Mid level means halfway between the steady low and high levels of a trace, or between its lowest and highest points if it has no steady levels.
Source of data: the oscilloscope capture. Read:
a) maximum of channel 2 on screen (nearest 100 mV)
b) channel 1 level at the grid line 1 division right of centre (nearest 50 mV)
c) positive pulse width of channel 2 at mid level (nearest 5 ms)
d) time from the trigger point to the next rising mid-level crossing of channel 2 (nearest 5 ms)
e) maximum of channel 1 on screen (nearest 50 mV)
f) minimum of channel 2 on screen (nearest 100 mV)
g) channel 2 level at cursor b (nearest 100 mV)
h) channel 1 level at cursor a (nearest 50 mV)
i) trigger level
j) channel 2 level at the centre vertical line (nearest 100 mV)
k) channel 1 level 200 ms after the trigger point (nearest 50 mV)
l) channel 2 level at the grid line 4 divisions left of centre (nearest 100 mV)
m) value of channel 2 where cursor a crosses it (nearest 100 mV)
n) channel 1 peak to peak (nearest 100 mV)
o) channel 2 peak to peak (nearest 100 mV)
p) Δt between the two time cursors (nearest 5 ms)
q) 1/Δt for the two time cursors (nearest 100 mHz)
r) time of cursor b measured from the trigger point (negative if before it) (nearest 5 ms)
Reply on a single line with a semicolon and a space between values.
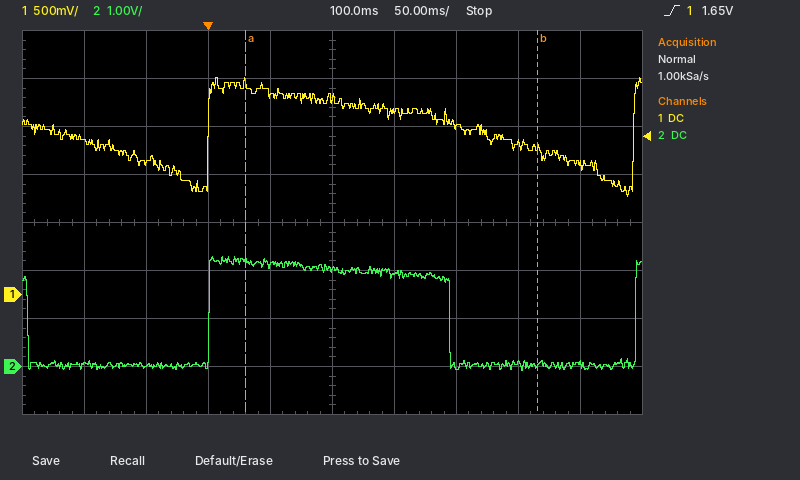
2.3 V; 1.90 V; 195 ms; 345 ms; 2.25 V; -100 mV; 0.0 V; 2.20 V; 1.65 V; 2.0 V; 1.75 V; 0.0 V; 2.2 V; 1.20 V; 2.4 V; 235 ms; 4.3 Hz; +265 ms
